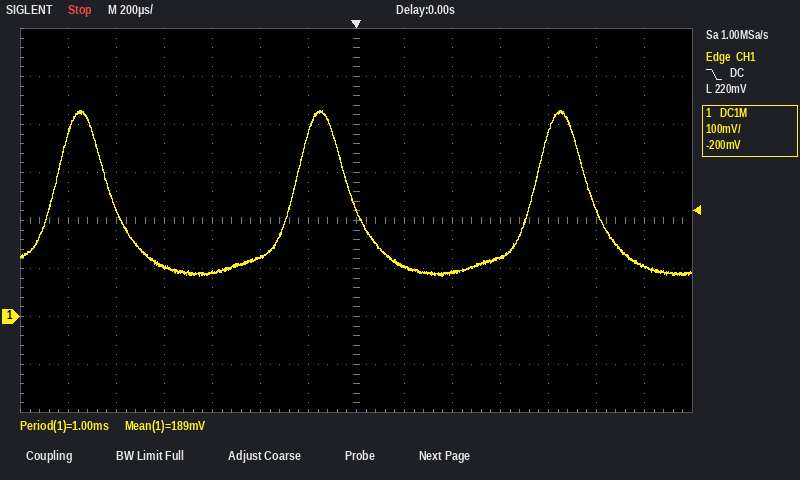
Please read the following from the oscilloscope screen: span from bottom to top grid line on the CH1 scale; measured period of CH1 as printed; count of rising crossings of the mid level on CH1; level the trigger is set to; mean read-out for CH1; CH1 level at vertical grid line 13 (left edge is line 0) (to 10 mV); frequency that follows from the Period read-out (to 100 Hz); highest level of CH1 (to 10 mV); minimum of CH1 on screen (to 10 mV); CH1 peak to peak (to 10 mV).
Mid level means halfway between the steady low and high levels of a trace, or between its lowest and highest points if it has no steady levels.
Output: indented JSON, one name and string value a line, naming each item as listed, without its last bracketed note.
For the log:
{
  "span from bottom to top grid line on the CH1 scale": "800 mV",
  "measured period of CH1 as printed": "1.00 ms",
  "count of rising crossings of the mid level on CH1": "3",
  "level the trigger is set to": "220 mV",
  "mean read-out for CH1": "189 mV",
  "CH1 level at vertical grid line 13 (left edge is line 0)": "100 mV",
  "frequency that follows from the Period read-out": "1.0 kHz",
  "highest level of CH1": "430 mV",
  "minimum of CH1 on screen": "80 mV",
  "CH1 peak to peak": "350 mV"
}
